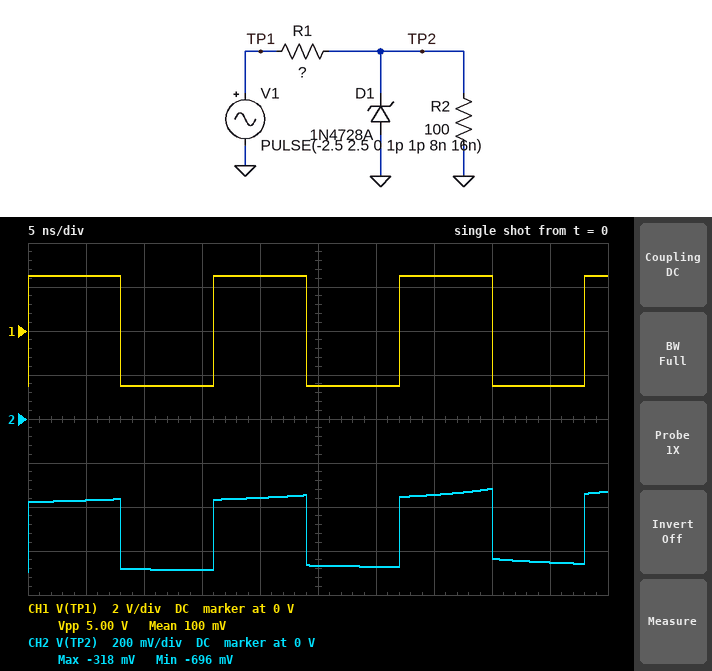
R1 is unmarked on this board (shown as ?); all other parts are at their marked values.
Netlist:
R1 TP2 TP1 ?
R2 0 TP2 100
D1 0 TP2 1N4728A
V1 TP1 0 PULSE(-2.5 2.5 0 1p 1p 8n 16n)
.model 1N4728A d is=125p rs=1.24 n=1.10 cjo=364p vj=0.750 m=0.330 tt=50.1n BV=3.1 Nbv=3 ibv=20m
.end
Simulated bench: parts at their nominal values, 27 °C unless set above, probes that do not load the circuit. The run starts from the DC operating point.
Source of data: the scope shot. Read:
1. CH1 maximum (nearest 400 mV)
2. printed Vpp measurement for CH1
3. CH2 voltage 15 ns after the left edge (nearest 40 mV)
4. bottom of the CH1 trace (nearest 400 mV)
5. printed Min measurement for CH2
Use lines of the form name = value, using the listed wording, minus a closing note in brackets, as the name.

CH1 maximum = 2.4 V
printed Vpp measurement for CH1 = 5.00 V
CH2 voltage 15 ns after the left edge = -680 mV
bottom of the CH1 trace = -2.4 V
printed Min measurement for CH2 = -696 mV
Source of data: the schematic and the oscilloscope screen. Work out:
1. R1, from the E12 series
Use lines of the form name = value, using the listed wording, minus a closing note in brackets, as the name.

R1, from the E12 series = 18 Ω
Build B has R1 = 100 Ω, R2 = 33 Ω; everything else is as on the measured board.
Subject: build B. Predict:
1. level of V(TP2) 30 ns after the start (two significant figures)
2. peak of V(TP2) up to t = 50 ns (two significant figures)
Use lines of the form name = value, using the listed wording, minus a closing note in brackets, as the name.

level of V(TP2) 30 ns after the start = -230 mV
peak of V(TP2) up to t = 50 ns = 250 mV
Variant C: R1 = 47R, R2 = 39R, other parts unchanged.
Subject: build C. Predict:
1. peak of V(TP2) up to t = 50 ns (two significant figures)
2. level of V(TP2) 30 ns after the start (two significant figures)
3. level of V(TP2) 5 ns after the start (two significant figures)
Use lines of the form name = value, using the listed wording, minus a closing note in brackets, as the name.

peak of V(TP2) up to t = 50 ns = 180 mV
level of V(TP2) 30 ns after the start = -530 mV
level of V(TP2) 5 ns after the start = -440 mV
